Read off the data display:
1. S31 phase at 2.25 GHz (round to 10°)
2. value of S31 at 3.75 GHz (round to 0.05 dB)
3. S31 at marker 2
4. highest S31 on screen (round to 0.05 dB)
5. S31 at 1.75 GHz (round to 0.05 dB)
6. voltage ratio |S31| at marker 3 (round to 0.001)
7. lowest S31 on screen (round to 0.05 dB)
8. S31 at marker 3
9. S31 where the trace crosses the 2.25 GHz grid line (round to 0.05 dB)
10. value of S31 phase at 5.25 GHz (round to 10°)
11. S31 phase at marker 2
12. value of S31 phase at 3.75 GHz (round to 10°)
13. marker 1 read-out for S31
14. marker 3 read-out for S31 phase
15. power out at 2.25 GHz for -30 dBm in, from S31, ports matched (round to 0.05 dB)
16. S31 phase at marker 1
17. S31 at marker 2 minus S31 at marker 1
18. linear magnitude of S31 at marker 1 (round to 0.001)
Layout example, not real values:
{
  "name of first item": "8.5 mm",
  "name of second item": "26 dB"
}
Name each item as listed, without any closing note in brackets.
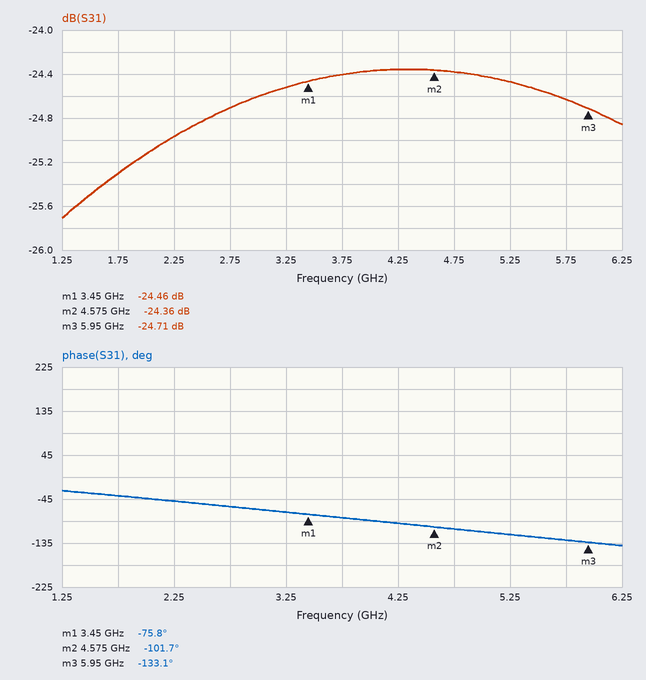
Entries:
{
  "S31 phase at 2.25 GHz": "-50°",
  "value of S31 at 3.75 GHz": "-24.40 dB",
  "S31 at marker 2": "-24.36 dB",
  "highest S31 on screen": "-24.35 dB",
  "S31 at 1.75 GHz": "-25.30 dB",
  "voltage ratio |S31| at marker 3": "0.058",
  "lowest S31 on screen": "-25.70 dB",
  "S31 at marker 3": "-24.71 dB",
  "S31 where the trace crosses the 2.25 GHz grid line": "-24.95 dB",
  "value of S31 phase at 5.25 GHz": "-120°",
  "S31 phase at marker 2": "-101.7°",
  "value of S31 phase at 3.75 GHz": "-80°",
  "marker 1 read-out for S31": "-24.46 dB",
  "marker 3 read-out for S31 phase": "-133.1°",
  "power out at 2.25 GHz for -30 dBm in, from S31, ports matched": "-54.95 dBm",
  "S31 phase at marker 1": "-75.8°",
  "S31 at marker 2 minus S31 at marker 1": "0.10 dB",
  "linear magnitude of S31 at marker 1": "0.060"
}
